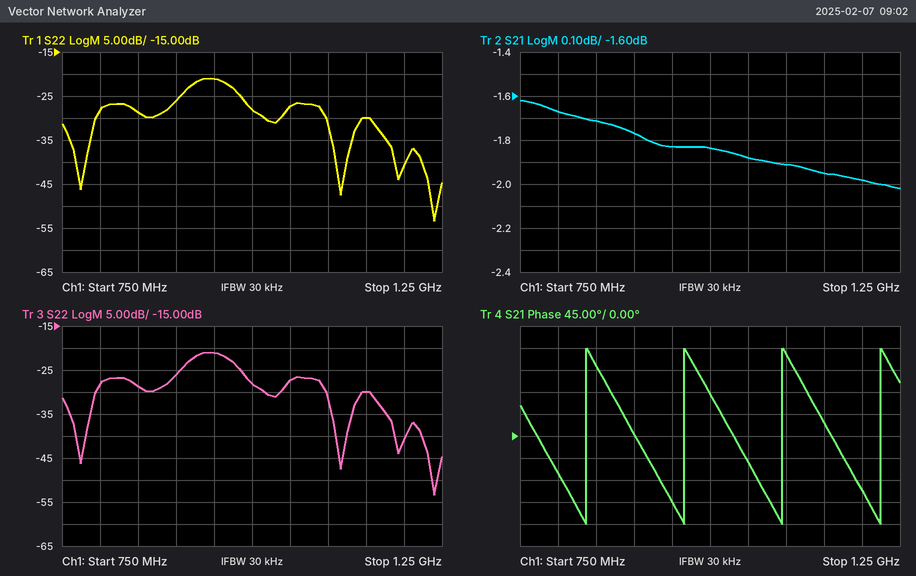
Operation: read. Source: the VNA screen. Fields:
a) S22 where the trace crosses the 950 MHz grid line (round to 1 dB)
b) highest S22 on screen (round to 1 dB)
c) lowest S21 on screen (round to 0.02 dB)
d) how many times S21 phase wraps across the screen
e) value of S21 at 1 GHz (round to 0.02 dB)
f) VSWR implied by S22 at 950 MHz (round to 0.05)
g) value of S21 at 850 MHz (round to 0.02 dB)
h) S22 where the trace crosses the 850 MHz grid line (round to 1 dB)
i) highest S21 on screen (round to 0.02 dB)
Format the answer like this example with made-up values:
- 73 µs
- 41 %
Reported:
- -21 dB
- -21 dB
- -2.02 dB
- 4
- -1.84 dB
- 1.20
- -1.72 dB
- -29 dB
- -1.62 dB
